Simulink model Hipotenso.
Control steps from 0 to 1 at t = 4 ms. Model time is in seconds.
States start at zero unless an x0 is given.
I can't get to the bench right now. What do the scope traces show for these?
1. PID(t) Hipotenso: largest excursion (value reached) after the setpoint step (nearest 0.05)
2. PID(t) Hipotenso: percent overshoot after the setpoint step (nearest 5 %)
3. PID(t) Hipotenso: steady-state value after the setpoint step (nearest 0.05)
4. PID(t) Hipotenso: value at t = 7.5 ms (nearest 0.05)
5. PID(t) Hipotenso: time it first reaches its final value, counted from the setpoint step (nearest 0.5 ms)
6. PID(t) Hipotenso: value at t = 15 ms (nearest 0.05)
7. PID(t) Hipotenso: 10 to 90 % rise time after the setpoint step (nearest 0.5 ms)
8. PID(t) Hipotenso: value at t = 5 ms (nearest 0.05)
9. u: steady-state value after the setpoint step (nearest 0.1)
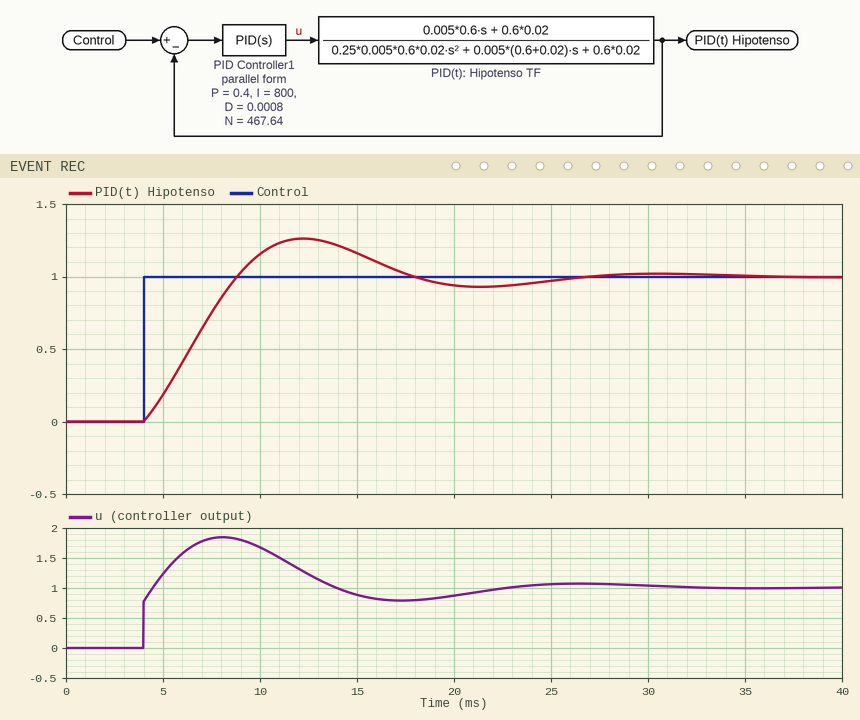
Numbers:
1.25
25 %
1.00
0.75
5.0 ms
1.15
3.5 ms
0.20
1.0
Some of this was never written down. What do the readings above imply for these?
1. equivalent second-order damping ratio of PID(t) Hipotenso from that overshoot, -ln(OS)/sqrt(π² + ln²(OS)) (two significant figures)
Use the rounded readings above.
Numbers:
0.40
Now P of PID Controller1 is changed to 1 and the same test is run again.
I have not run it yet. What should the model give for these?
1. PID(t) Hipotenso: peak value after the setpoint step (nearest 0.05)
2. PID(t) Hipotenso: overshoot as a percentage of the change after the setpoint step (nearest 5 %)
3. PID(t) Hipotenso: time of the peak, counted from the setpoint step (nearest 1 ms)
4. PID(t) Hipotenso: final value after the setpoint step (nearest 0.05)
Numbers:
1.15
15 %
8 ms
1.00
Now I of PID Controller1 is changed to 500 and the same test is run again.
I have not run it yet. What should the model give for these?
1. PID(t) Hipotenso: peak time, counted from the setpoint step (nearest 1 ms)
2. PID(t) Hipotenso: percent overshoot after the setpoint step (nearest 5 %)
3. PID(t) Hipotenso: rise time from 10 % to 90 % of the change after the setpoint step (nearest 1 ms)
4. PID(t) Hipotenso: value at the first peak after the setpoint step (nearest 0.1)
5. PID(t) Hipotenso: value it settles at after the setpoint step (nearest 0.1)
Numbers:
11 ms
20 %
5 ms
1.2
1.0
